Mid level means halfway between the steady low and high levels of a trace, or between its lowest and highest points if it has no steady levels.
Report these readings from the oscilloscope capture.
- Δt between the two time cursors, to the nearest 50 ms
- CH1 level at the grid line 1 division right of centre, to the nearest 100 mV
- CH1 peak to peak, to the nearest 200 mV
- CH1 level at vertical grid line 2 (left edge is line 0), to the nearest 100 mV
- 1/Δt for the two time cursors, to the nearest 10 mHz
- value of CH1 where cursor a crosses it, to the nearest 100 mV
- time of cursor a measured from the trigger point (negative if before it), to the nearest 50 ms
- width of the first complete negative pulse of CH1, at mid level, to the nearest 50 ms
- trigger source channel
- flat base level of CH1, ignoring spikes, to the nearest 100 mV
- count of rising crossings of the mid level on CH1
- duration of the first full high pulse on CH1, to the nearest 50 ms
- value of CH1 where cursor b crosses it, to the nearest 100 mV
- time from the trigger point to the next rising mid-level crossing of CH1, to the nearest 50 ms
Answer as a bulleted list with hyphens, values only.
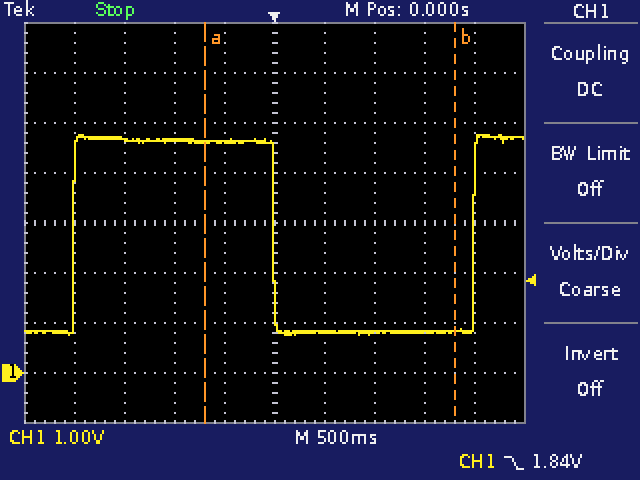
- 2.50 s
- 800 mV
- 4.0 V
- 4.7 V
- 400 mHz
- 4.6 V
- -700 ms
- 2.00 s
- CH1
- 800 mV
- 2
- 2.00 s
- 800 mV
- 2.00 s
